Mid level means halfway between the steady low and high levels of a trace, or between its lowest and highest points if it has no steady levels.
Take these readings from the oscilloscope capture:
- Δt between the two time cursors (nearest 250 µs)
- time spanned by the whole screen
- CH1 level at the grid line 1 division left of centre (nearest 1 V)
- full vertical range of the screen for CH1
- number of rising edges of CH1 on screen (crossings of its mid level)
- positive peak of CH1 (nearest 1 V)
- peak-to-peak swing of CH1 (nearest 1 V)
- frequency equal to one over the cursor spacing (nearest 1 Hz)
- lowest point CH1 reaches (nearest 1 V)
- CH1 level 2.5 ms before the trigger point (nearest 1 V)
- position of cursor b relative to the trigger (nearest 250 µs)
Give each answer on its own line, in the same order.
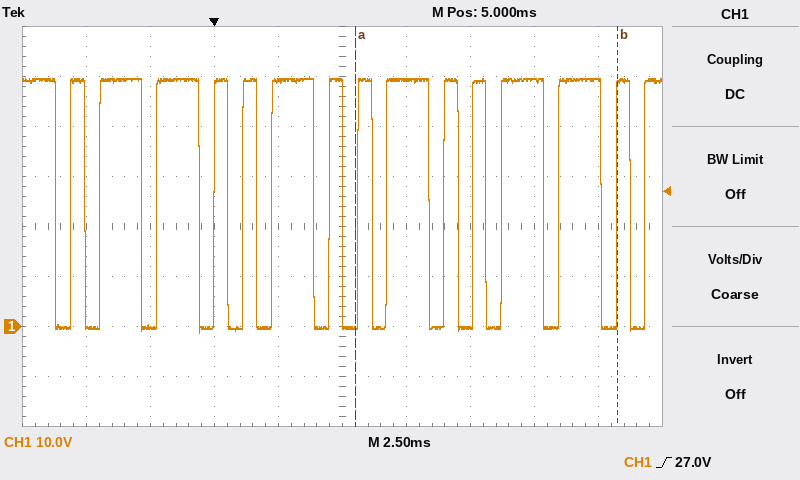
10.25 ms
25 ms
49 V
80 V
15
50 V
51 V
98 Hz
-1 V
0 V
+15.75 ms
